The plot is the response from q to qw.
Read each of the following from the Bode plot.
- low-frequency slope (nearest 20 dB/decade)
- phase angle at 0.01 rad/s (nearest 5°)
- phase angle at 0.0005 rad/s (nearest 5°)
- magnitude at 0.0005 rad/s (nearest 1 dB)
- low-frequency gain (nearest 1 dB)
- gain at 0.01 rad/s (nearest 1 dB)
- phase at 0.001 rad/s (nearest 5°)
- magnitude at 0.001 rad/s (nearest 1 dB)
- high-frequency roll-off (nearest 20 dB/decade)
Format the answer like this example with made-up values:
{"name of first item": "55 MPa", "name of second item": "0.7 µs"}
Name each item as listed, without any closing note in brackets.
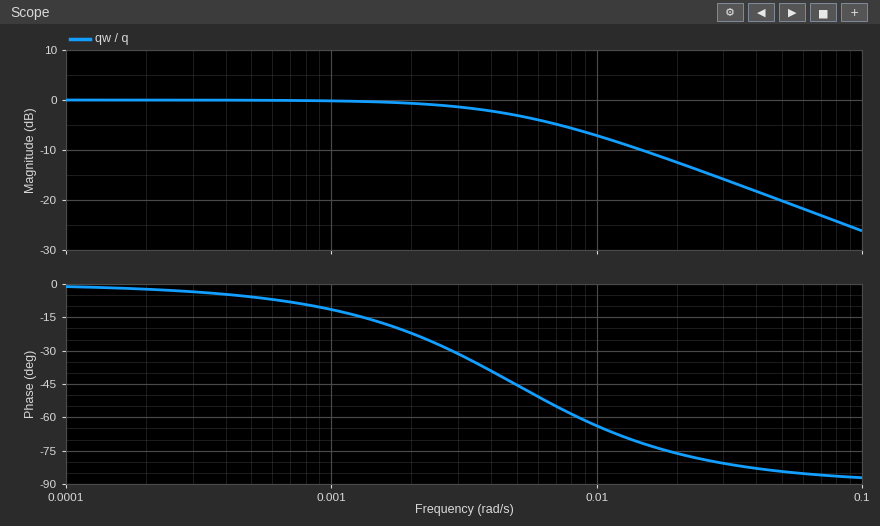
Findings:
{"low-frequency slope": "0 dB/decade", "phase angle at 0.01 rad/s": "-65°", "phase angle at 0.0005 rad/s": "-5°", "magnitude at 0.0005 rad/s": "0 dB", "low-frequency gain": "0 dB", "gain at 0.01 rad/s": "-7 dB", "phase at 0.001 rad/s": "-10°", "magnitude at 0.001 rad/s": "0 dB", "high-frequency roll-off": "-20 dB/decade"}
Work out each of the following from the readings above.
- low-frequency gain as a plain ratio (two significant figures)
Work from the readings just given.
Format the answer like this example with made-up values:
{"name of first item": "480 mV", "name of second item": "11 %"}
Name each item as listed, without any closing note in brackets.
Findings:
{"low-frequency gain as a plain ratio": "1.0"}
